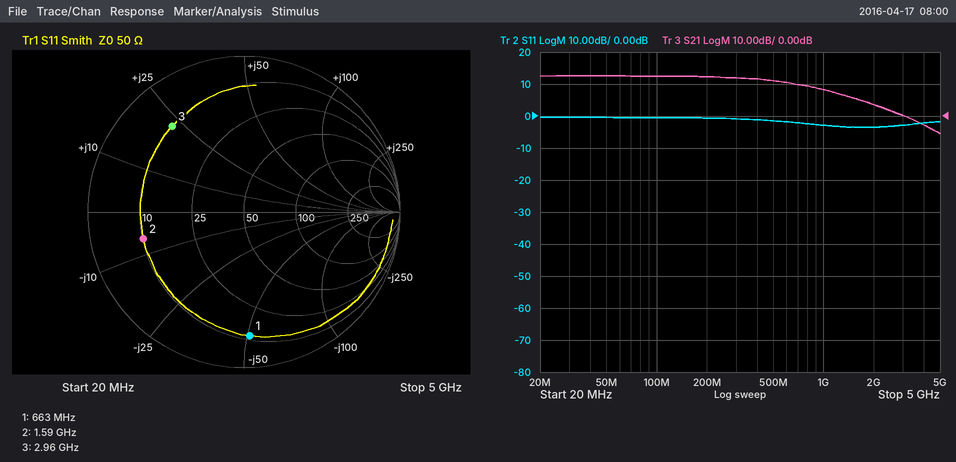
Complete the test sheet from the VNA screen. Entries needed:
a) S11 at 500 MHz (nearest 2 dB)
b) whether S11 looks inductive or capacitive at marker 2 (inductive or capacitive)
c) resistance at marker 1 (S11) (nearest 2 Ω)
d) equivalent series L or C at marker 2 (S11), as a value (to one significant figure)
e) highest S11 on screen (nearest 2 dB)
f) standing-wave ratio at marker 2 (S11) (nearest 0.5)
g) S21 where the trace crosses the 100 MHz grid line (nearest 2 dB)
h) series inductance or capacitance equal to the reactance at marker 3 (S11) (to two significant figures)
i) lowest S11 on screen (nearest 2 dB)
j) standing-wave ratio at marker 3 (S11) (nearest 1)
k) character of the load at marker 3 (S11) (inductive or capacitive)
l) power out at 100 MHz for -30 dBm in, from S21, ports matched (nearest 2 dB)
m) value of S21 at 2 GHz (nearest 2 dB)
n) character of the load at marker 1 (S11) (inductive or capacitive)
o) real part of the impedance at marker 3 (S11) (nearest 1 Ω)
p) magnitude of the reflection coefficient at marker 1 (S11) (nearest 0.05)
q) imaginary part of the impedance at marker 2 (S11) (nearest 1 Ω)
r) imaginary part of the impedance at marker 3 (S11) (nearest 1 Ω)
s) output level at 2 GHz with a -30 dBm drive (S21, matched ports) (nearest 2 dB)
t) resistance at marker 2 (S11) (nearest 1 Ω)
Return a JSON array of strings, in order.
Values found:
["-2 dB", "capacitive", "12 Ω", "20 pF", "0 dB", "5.0", "12 dB", "1.2 nH", "-4 dB", "6", "inductive", "-18 dBm", "4 dB", "capacitive", "10 Ω", "0.80", "-6 Ω", "+23 Ω", "-26 dBm", "10 Ω"]
